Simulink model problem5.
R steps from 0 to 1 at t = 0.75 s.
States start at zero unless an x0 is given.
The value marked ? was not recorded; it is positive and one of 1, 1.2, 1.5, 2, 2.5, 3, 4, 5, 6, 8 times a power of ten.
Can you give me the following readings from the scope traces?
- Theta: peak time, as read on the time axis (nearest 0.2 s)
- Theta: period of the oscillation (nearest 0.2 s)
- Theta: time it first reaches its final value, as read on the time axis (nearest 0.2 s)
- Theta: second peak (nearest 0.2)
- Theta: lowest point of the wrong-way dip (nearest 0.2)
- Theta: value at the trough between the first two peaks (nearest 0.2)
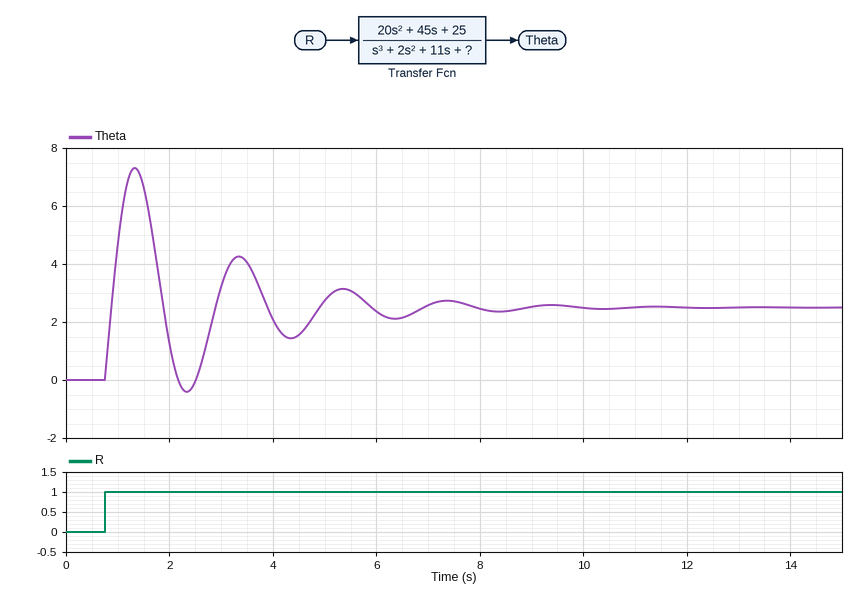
1.4 s
2.0 s
0.8 s
4.2
-0.4
-0.4
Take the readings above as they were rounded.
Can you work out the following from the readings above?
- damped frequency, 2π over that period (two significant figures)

3.1 rad/s
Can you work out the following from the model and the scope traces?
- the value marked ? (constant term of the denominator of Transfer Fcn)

10
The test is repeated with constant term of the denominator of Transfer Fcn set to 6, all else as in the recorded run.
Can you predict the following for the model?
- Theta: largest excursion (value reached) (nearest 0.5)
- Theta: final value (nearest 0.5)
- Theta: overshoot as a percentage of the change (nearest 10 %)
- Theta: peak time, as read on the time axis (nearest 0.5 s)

7.5
4.0
80 %
1.5 s
